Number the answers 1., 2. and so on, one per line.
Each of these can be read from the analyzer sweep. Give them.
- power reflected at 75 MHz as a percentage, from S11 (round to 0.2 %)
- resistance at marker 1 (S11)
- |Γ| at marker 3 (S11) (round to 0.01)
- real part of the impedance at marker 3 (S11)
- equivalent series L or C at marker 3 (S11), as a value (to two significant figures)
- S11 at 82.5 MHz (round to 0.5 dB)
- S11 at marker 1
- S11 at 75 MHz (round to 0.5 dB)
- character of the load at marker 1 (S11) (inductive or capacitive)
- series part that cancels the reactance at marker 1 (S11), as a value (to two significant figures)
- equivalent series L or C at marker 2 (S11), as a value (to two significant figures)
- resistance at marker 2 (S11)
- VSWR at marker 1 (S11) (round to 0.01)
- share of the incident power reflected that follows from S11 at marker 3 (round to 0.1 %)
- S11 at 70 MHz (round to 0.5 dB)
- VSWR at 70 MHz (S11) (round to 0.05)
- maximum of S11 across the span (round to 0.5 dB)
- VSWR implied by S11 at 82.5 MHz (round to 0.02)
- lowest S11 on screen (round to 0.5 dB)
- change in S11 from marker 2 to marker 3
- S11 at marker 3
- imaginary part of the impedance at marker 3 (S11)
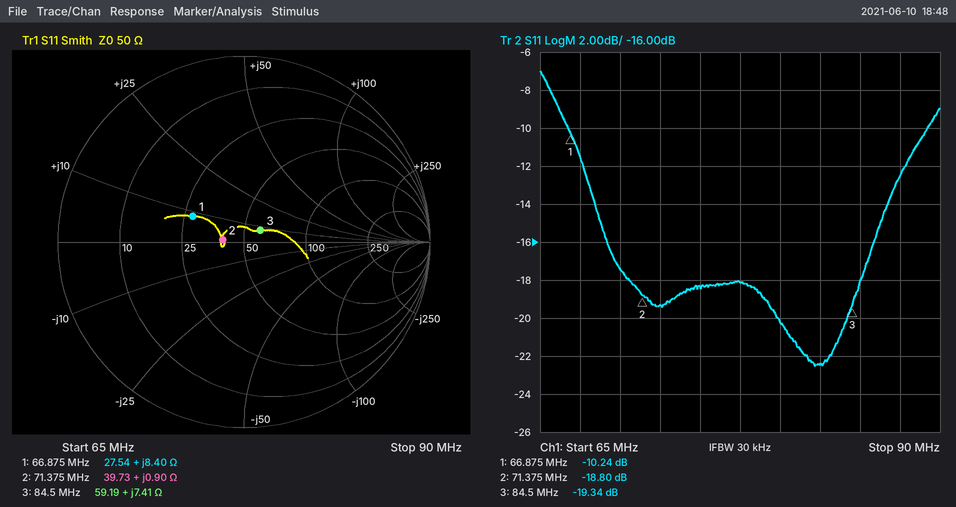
1. 1.4 %
2. 27.54 Ω
3. 0.11
4. 59.19 Ω
5. 14 nH
6. -22.5 dB
7. -10.24 dB
8. -18.5 dB
9. inductive
10. 280 pF
11. 2.0 nH
12. 39.73 Ω
13. 1.89
14. 1.2 %
15. -17.5 dB
16. 1.30
17. -7.0 dB
18. 1.16
19. -22.5 dB
20. -0.54 dB
21. -19.34 dB
22. +7.41 Ω
